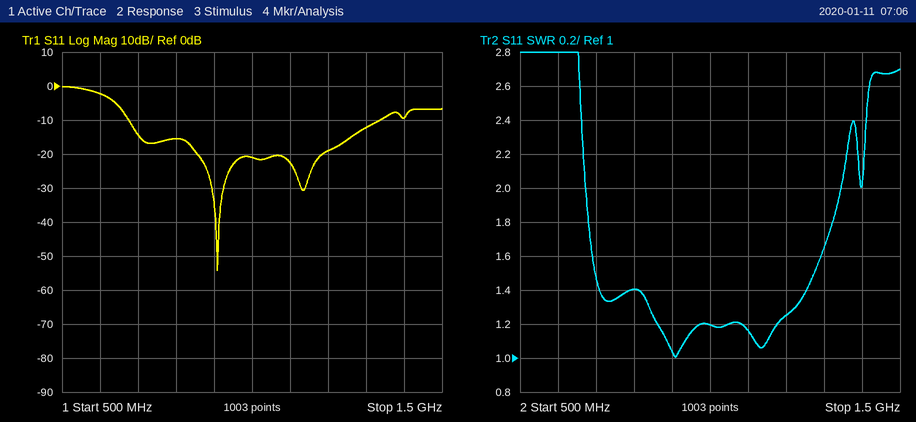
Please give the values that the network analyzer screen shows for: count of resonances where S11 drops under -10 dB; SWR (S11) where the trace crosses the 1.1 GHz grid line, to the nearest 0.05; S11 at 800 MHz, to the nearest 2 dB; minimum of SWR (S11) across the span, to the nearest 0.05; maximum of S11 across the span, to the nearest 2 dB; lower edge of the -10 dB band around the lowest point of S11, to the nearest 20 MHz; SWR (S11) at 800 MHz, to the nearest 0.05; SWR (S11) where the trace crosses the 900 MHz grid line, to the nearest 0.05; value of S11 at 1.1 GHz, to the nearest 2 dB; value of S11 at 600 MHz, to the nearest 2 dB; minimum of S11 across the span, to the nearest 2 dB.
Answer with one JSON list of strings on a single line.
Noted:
["2", "1.15", "-16 dB", "1.00", "0 dB", "680 MHz", "1.40", "1.05", "-22 dB", "-2 dB", "-54 dB"]
